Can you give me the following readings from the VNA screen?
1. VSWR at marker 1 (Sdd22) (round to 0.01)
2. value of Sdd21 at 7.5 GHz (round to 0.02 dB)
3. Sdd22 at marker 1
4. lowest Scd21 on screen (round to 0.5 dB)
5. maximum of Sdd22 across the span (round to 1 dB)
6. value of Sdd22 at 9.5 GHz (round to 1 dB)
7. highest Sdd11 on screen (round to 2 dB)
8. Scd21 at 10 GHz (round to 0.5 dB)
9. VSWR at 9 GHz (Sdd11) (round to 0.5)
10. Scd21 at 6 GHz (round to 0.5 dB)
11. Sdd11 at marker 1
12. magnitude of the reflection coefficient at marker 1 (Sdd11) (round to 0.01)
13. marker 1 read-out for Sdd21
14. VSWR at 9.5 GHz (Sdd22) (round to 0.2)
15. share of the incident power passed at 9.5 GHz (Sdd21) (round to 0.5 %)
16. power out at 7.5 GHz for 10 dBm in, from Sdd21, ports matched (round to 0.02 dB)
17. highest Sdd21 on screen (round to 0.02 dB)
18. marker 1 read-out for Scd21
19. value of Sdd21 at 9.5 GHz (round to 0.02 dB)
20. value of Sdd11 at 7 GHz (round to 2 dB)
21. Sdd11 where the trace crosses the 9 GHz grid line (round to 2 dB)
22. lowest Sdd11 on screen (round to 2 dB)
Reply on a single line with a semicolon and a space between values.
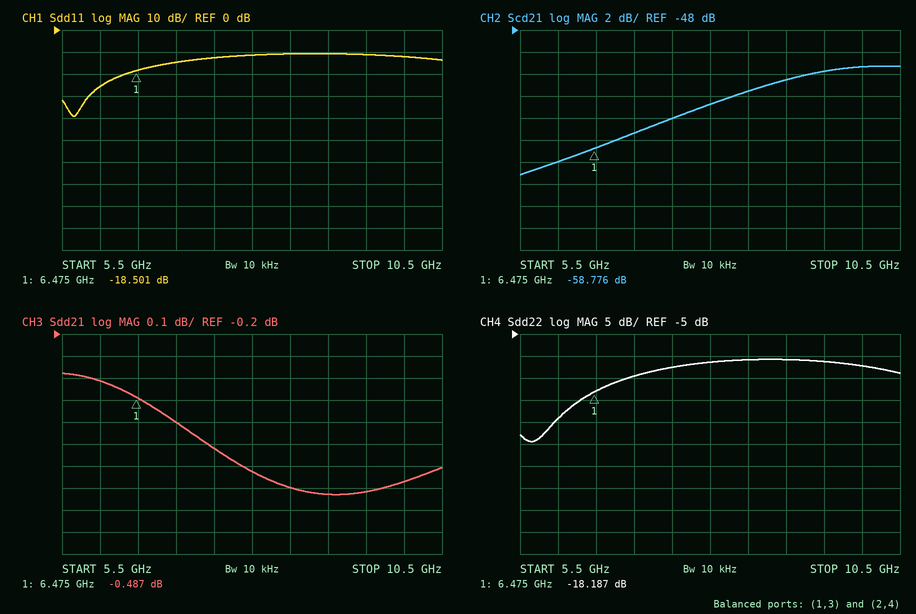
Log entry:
1.28; -0.72 dB; -18.187 dB; -61.0 dB; -11 dB; -11 dB; -10 dB; -51.5 dB; 2.0; -60.0 dB; -18.501 dB; 0.12; -0.487 dB; 1.8; 81.0 %; 9.28 dBm; -0.38 dB; -58.776 dB; -0.92 dB; -14 dB; -10 dB; -40 dB
